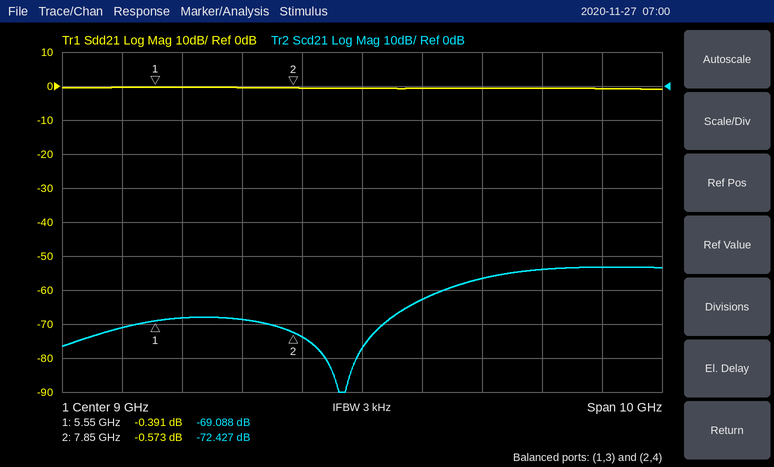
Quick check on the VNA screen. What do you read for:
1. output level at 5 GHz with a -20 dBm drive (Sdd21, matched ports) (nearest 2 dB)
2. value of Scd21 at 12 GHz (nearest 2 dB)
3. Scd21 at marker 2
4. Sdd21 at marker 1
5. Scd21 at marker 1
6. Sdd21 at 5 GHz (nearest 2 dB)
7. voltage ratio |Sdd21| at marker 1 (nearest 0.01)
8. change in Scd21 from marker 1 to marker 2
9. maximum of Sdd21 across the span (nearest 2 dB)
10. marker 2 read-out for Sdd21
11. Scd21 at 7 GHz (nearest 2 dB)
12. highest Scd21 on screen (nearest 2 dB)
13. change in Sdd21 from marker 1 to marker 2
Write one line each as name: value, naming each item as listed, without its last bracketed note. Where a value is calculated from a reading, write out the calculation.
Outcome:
output level at 5 GHz with a -20 dBm drive (Sdd21, matched ports): -20 dBm + (0 dB) = -20 dBm
value of Scd21 at 12 GHz: -54 dB
Scd21 at marker 2: -72.427 dB
Sdd21 at marker 1: -0.391 dB
Scd21 at marker 1: -69.088 dB
Sdd21 at 5 GHz: 0 dB
voltage ratio |Sdd21| at marker 1: 10^(-0.391/20) ≈ 0.96
change in Scd21 from marker 1 to marker 2: -72.427 − (-69.088) = -3.339 dB
maximum of Sdd21 across the span: 0 dB
marker 2 read-out for Sdd21: -0.573 dB
Scd21 at 7 GHz: -68 dB
highest Scd21 on screen: -54 dB
change in Sdd21 from marker 1 to marker 2: -0.573 − (-0.391) = -0.182 dB
